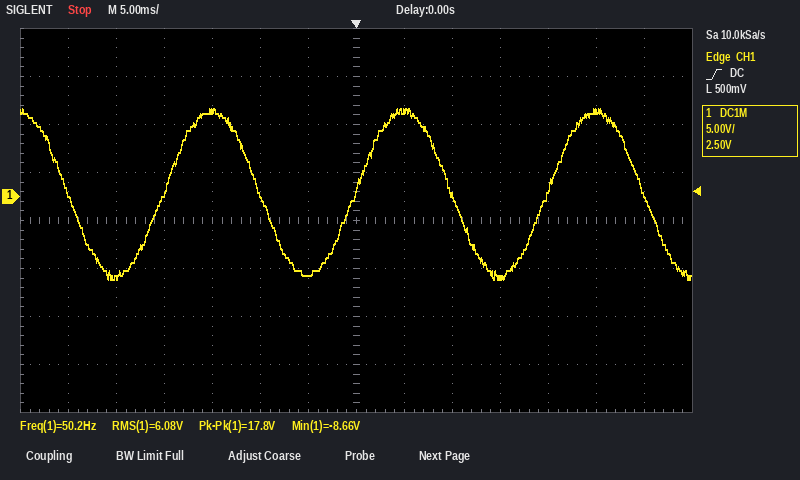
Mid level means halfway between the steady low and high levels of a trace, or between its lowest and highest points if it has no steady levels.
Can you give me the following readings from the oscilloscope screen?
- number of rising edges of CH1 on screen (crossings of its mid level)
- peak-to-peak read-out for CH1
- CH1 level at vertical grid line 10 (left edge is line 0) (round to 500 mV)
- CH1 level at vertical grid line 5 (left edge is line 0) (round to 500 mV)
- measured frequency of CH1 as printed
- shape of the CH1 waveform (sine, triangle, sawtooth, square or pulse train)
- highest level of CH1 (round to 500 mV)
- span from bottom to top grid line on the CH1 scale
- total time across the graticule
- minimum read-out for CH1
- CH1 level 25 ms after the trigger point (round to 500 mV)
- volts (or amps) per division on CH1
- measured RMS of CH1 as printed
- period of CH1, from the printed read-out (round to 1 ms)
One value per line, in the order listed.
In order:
3
17.8 V
-8.5 V
0.0 V
50.2 Hz
sine
9.0 V
40 V
70 ms
-8.66 V
9.0 V
5 V
6.08 V
20 ms
